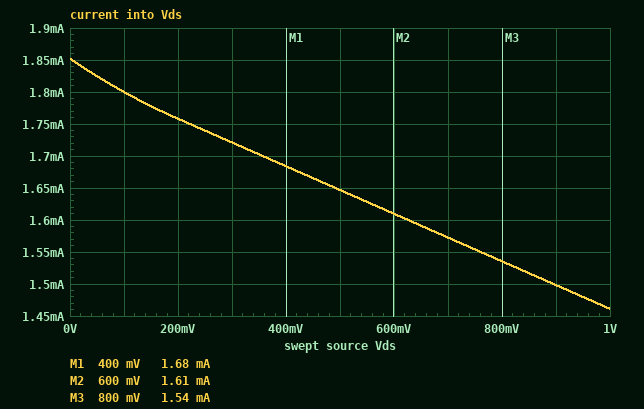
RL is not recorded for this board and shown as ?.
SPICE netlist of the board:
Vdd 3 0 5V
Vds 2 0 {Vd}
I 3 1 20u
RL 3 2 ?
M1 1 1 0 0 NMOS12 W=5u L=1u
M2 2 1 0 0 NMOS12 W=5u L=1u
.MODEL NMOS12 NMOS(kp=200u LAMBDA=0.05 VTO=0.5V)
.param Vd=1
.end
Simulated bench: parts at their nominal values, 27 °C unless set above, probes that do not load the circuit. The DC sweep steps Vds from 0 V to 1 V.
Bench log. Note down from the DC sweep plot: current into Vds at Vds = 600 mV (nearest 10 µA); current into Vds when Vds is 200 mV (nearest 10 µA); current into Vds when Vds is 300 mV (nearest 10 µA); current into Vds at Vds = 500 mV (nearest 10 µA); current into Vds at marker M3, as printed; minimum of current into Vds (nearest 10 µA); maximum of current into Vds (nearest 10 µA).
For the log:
1.61 mA
1.76 mA
1.72 mA
1.65 mA
1.54 mA
1.46 mA
1.85 mA
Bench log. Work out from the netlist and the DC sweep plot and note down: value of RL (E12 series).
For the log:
2.7 kΩ
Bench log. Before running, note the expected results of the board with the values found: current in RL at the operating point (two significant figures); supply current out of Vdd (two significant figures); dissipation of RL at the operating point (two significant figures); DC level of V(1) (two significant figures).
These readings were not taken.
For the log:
1.5 mA
1.5 mA
5.9 mW
700 mV
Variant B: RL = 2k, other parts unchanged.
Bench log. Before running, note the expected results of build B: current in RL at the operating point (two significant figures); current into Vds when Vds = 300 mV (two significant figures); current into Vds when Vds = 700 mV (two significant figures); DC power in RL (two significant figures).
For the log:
2.0 mA
2.3 mA
2.1 mA
8.0 mW
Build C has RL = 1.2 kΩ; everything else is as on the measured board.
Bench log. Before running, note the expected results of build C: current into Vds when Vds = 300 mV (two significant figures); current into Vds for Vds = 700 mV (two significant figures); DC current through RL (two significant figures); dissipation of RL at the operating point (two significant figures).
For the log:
3.9 mA
3.6 mA
3.3 mA
13 mW
